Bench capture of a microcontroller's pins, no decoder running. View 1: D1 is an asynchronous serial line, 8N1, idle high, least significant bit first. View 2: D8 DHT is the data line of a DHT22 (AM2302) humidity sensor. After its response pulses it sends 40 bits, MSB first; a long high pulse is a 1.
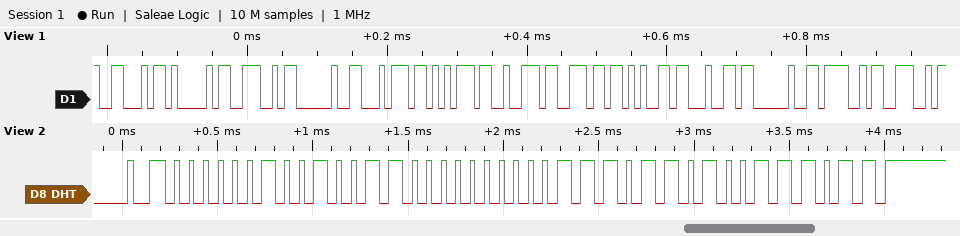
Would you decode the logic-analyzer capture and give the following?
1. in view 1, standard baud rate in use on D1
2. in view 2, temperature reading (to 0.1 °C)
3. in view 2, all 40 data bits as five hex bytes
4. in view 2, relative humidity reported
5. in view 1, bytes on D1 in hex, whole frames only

115200 baud
23.7 °C
02 4C 00 ED 3B
58.8 %
0x46 0x41 0x4E 0x20 0x74 0x75 0x72 0x6E 0x65 0x64 0x20 0x4F 0x4E
